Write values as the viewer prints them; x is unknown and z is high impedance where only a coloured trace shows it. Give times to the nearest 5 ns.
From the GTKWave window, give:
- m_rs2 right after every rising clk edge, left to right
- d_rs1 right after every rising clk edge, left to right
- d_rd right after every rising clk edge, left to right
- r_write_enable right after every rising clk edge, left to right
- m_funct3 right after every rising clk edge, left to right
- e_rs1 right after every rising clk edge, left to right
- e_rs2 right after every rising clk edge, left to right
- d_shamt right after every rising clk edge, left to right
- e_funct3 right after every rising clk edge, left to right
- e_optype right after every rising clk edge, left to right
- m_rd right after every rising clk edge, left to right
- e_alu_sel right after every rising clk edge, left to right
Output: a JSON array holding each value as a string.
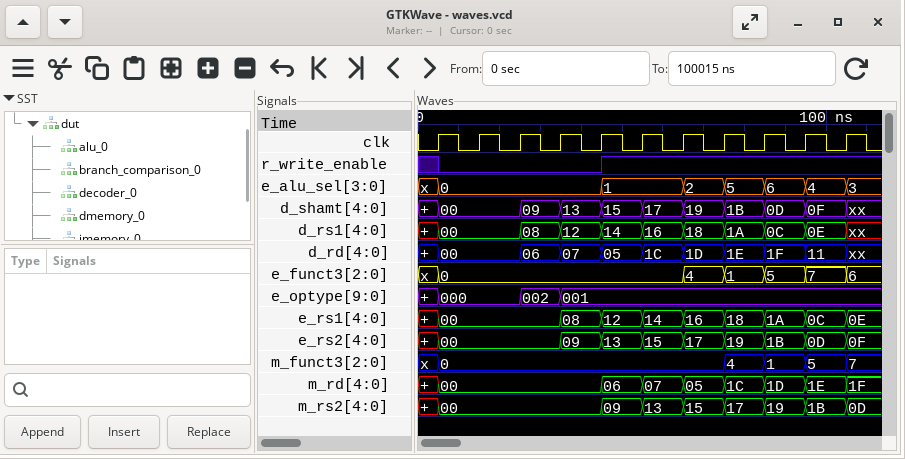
["00, 00, 00, 00, 09, 13, 15, 17, 19, 1B, 0D", "00, 00, 08, 12, 14, 16, 18, 1A, 0C, 0E, xx", "00, 00, 06, 07, 05, 1C, 1D, 1E, 1F, 11, xx", "0 0 0 0 1 1 1 1 1 1 1", "0, 0, 0, 0, 0, 0, 0, 4, 1, 5, 7", "00, 00, 00, 08, 12, 14, 16, 18, 1A, 0C, 0E", "00, 00, 00, 09, 13, 15, 17, 19, 1B, 0D, 0F", "00, 00, 09, 13, 15, 17, 19, 1B, 0D, 0F, xx", "0, 0, 0, 0, 0, 0, 4, 1, 5, 7, 6", "000, 000, 002, 001, 001, 001, 001, 001, 001, 001, 001", "00, 00, 00, 00, 06, 07, 05, 1C, 1D, 1E, 1F", "0, 0, 0, 0, 1, 1, 2, 5, 6, 4, 3"]
